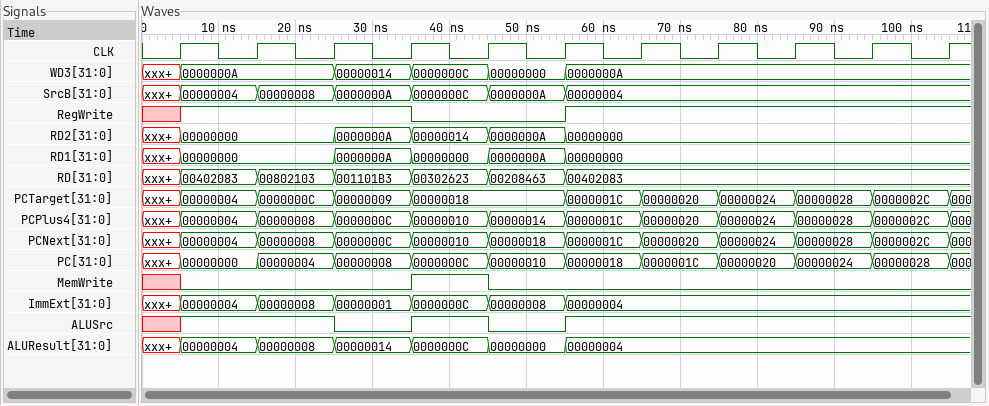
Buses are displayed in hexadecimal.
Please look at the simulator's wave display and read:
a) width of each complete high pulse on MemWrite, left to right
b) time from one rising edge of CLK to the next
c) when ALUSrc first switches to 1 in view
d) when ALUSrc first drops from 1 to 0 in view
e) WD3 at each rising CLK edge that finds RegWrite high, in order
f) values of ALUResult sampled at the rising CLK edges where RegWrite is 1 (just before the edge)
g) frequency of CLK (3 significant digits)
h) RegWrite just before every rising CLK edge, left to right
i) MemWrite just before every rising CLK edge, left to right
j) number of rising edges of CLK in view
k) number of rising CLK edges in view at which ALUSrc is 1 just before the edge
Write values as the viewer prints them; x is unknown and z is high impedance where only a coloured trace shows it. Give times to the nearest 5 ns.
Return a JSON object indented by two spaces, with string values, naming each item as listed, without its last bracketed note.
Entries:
{
  "width of each complete high pulse on MemWrite, left to right": "10 ns",
  "time from one rising edge of CLK to the next": "10 ns",
  "when ALUSrc first switches to 1 in view": "5 ns",
  "when ALUSrc first drops from 1 to 0 in view": "25 ns",
  "WD3 at each rising CLK edge that finds RegWrite high, in order": "0000000A, 0000000A, 00000014, 0000000A, 0000000A, 0000000A, 0000000A, 0000000A",
  "values of ALUResult sampled at the rising CLK edges where RegWrite is 1": "00000004, 00000008, 00000014, 00000004, 00000004, 00000004, 00000004, 00000004",
  "frequency of CLK": "100 MHz",
  "RegWrite just before every rising CLK edge, left to right": "x 1 1 1 0 0 1 1 1 1 1",
  "MemWrite just before every rising CLK edge, left to right": "x 0 0 0 1 0 0 0 0 0 0",
  "number of rising edges of CLK in view": "11",
  "number of rising CLK edges in view at which ALUSrc is 1 just before the edge": "8"
}
